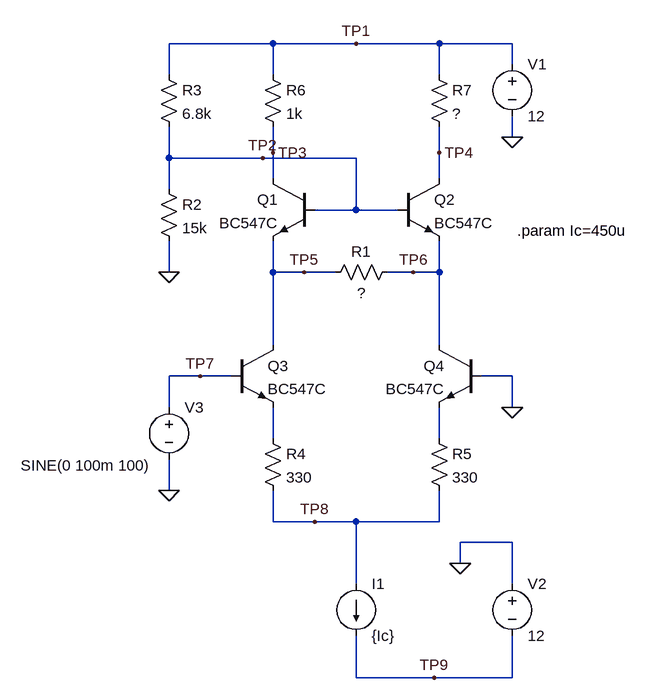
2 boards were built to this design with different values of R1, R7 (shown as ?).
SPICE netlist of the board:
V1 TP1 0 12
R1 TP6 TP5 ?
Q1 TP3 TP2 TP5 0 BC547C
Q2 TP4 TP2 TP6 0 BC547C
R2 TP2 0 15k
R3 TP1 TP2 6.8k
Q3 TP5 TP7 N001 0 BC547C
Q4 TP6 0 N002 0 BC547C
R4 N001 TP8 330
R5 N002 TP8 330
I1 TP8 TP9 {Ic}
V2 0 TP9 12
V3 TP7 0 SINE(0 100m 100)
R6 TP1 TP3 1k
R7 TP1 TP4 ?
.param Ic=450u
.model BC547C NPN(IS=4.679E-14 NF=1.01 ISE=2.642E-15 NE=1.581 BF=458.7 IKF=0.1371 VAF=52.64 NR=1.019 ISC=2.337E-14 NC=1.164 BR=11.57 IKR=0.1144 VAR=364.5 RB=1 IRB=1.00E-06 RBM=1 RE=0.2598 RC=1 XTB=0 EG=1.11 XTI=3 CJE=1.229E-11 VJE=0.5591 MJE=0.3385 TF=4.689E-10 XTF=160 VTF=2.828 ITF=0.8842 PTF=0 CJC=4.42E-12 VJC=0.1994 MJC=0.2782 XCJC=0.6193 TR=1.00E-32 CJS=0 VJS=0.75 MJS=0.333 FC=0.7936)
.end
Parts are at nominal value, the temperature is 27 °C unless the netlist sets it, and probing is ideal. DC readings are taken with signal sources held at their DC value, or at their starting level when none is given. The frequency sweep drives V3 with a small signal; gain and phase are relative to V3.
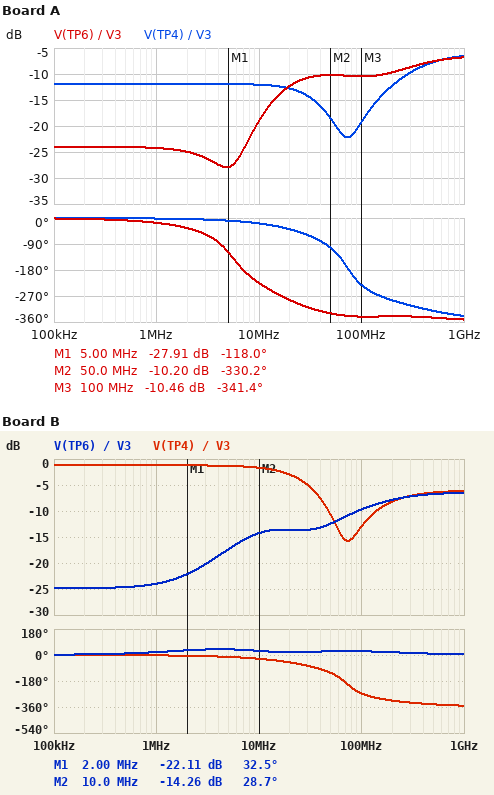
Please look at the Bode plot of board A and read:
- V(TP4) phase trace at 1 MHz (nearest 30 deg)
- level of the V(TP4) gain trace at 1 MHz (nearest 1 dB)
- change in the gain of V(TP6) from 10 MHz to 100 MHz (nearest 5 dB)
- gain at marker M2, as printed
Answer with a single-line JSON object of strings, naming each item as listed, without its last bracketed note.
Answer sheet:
{"V(TP4) phase trace at 1 MHz": "0 deg", "level of the V(TP4) gain trace at 1 MHz": "-12 dB", "change in the gain of V(TP6) from 10 MHz to 100 MHz": "10 dB", "gain at marker M2, as printed": "-10.20 dB"}
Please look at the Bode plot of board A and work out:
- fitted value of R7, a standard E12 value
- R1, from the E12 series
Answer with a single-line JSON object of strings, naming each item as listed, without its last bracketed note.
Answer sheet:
{"fitted value of R7, a standard E12 value": "470 Ω", "R1, from the E12 series": "220 Ω"}
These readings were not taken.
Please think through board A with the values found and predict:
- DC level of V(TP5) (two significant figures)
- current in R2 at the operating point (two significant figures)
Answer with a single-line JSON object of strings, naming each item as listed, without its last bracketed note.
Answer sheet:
{"DC level of V(TP5)": "7.7 V", "current in R2 at the operating point": "550 µA"}
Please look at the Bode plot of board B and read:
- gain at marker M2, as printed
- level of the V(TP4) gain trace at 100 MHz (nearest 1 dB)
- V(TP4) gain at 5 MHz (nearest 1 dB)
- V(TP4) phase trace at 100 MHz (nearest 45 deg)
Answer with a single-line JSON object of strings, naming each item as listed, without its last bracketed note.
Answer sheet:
{"gain at marker M2, as printed": "-14.26 dB", "level of the V(TP4) gain trace at 100 MHz": "-13 dB", "V(TP4) gain at 5 MHz": "-1 dB", "V(TP4) phase trace at 100 MHz": "-270 deg"}
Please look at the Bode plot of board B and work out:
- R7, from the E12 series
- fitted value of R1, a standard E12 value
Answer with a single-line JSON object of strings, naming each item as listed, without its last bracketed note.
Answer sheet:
{"R7, from the E12 series": "1.8 kΩ", "fitted value of R1, a standard E12 value": "180 Ω"}
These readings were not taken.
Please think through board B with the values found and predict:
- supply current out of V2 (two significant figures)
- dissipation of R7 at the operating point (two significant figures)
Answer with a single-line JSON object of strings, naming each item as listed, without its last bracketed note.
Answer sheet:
{"supply current out of V2": "450 µA", "dissipation of R7 at the operating point": "90 µW"}
